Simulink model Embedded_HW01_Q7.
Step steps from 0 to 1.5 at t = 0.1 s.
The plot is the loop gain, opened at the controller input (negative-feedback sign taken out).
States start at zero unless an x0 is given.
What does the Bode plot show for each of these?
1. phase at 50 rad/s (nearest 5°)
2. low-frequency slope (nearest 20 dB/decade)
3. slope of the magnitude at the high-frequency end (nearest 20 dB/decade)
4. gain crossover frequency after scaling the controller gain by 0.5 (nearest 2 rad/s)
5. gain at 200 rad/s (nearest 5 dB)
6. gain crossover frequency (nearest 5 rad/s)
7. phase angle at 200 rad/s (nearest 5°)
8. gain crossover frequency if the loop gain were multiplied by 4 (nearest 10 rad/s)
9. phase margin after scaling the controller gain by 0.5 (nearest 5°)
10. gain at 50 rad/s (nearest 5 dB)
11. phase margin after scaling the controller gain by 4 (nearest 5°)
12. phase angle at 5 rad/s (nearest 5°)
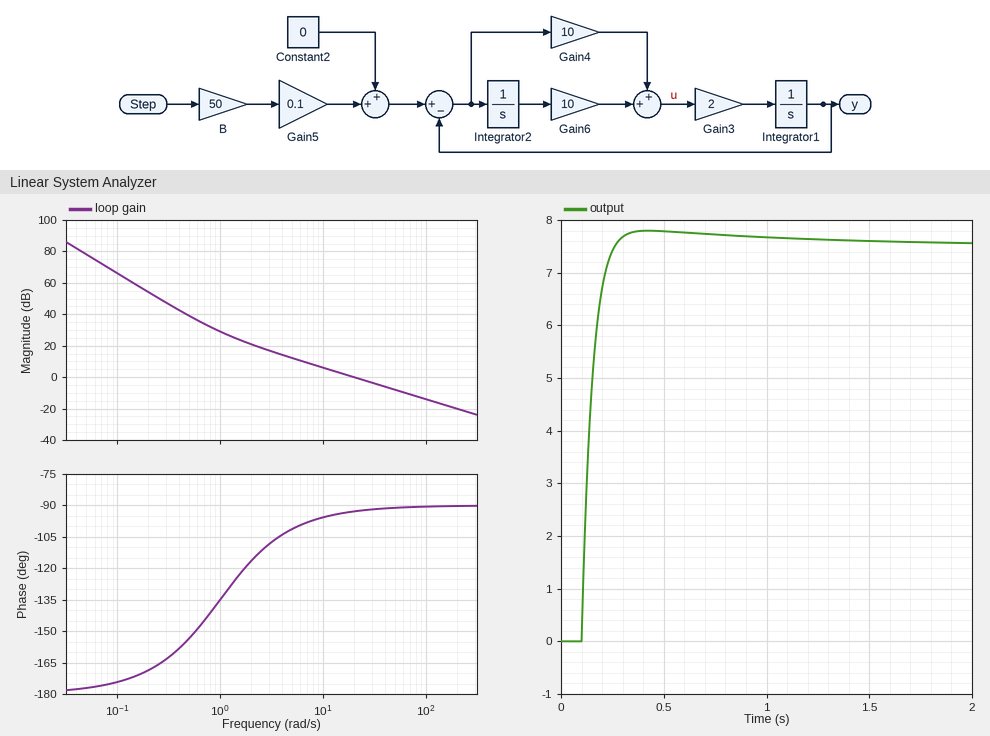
-90°
-40 dB/decade
-20 dB/decade
10 rad/s
-20 dB
20 rad/s
-90°
80 rad/s
85°
-10 dB
90°
-100°
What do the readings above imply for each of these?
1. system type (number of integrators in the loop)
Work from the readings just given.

2
